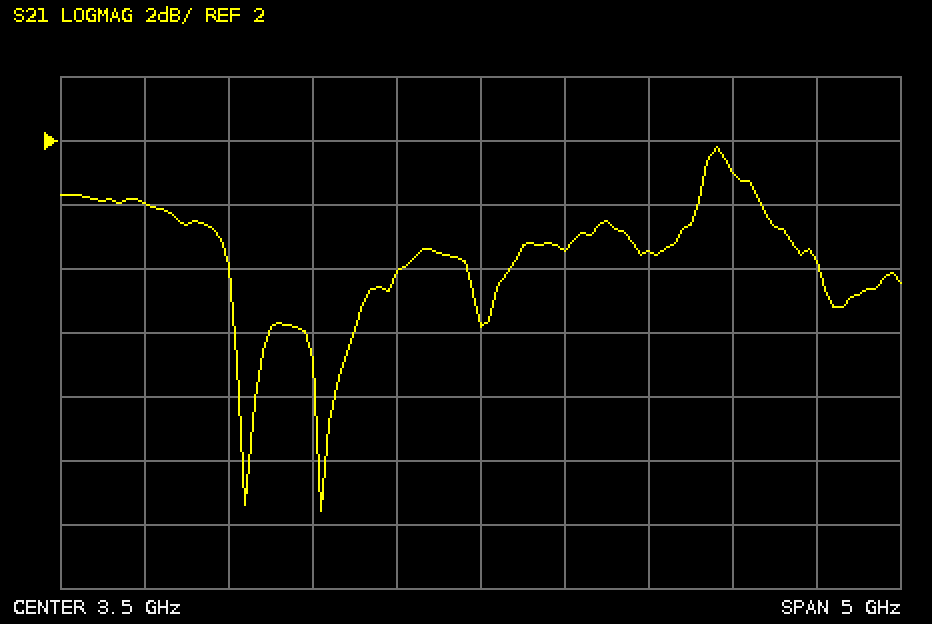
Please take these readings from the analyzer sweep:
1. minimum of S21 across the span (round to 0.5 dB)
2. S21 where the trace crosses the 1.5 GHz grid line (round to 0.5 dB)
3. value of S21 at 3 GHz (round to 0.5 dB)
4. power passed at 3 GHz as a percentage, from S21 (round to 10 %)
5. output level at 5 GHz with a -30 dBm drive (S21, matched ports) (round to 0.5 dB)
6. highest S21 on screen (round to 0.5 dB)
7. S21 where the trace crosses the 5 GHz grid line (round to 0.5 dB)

-9.5 dB
0.0 dB
-2.0 dB
60 %
-29.0 dBm
2.0 dB
1.0 dB
